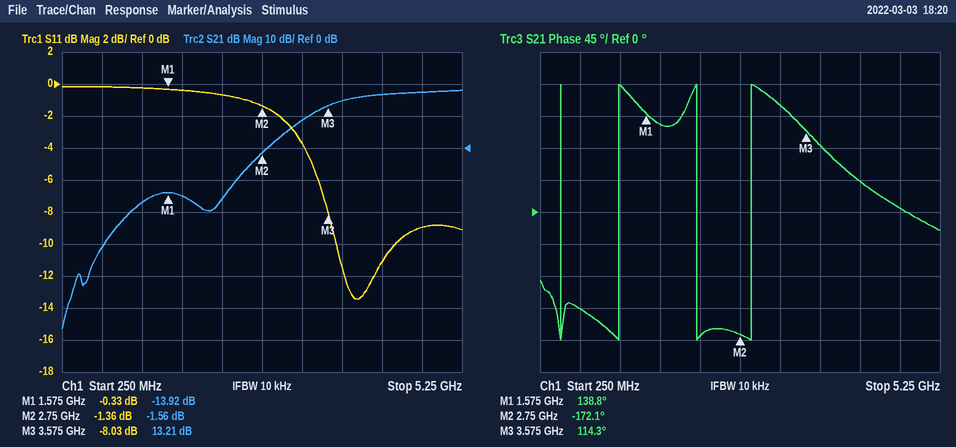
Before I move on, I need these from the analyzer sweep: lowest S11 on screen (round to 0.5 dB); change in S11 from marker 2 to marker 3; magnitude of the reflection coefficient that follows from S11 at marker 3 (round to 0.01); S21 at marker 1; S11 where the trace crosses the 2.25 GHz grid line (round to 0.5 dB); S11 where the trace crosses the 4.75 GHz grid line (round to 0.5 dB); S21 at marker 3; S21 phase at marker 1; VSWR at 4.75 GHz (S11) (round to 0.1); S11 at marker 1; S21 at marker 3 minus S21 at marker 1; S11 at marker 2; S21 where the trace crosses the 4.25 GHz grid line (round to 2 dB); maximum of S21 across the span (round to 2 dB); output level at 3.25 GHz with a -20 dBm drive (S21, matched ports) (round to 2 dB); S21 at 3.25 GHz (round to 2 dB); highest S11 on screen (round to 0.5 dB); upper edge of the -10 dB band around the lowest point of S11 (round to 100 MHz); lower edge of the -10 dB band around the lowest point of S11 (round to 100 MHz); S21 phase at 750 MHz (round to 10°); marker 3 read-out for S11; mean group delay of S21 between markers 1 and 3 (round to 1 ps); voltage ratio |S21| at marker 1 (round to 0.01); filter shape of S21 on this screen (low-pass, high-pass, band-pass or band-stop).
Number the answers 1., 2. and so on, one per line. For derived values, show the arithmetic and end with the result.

1. -13.5 dB
2. -8.03 − (-1.36) = -6.67 dB
3. 10^(-8.03/20) ≈ 0.40
4. -13.92 dB
5. -0.5 dB
6. -9.0 dB
7. 13.21 dB
8. 138.8°
9. |Γ| = 10^(-9/20) = 0.3548; VSWR = (1 + 0.3548)/(1 − 0.3548) ≈ 2.1
10. -0.33 dB
11. 13.21 − (-13.92) = 27.13 dB
12. -1.36 dB
13. 16 dB
14. 18 dB
15. -20 dBm + (8 dB) = -12 dBm
16. 8 dB
17. 0.0 dB
18. 4.4 GHz
19. 3.7 GHz
20. -140°
21. -8.03 dB
22. −(114.3° − (138.8°))/(360° × 2 GHz) ≈ 34 ps
23. 10^(-13.92/20) ≈ 0.20
24. high-pass
